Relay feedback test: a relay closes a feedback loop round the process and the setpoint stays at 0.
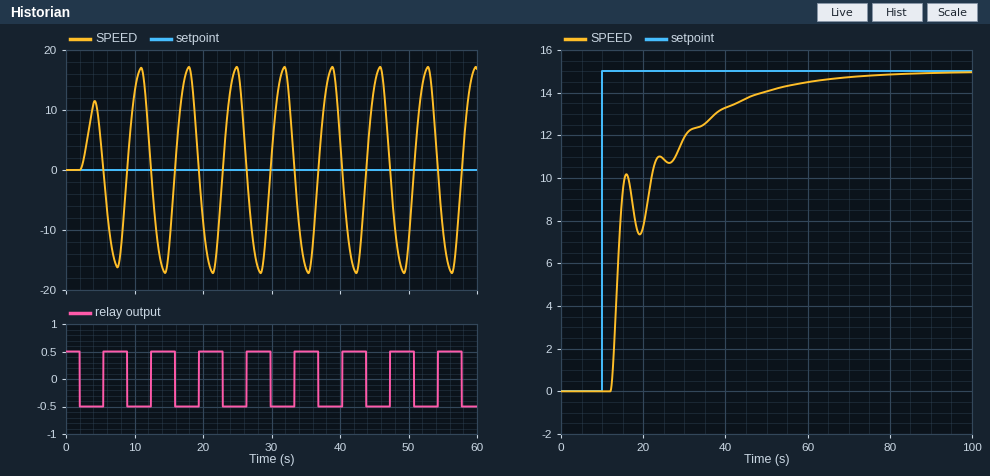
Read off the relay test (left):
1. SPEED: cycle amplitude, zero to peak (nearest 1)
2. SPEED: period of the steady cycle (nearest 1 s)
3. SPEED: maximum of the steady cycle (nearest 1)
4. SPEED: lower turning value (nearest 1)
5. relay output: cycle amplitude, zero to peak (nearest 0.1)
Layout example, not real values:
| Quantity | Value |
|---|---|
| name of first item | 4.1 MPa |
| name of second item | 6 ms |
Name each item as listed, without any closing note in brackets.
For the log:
| Quantity | Value |
|---|---|
| SPEED: cycle amplitude, zero to peak | 17 |
| SPEED: period of the steady cycle | 7 s |
| SPEED: maximum of the steady cycle | 17 |
| SPEED: lower turning value | -17 |
| relay output: cycle amplitude, zero to peak | 0.5 |
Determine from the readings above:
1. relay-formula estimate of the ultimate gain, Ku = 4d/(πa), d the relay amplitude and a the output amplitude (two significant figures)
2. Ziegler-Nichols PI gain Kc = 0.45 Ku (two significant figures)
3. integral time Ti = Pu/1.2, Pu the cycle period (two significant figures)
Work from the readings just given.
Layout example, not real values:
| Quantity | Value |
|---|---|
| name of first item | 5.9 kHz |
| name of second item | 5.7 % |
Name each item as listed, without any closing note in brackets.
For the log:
| Quantity | Value |
|---|---|
| relay-formula estimate of the ultimate gain, Ku = 4d/(πa), d the relay amplitude and a the output amplitude | 0.037 |
| Ziegler-Nichols PI gain Kc = 0.45 Ku | 0.017 |
| integral time Ti = Pu/1.2, Pu the cycle period | 5.8 s |
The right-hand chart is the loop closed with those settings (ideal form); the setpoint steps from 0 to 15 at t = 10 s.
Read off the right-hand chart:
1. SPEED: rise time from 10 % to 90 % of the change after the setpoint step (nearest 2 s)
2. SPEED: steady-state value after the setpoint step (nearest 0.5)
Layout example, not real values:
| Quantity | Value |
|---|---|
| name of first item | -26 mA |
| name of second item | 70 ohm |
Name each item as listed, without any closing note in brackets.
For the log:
| Quantity | Value |
|---|---|
| SPEED: rise time from 10 % to 90 % of the change after the setpoint step | 30 s |
| SPEED: steady-state value after the setpoint step | 15.0 |
